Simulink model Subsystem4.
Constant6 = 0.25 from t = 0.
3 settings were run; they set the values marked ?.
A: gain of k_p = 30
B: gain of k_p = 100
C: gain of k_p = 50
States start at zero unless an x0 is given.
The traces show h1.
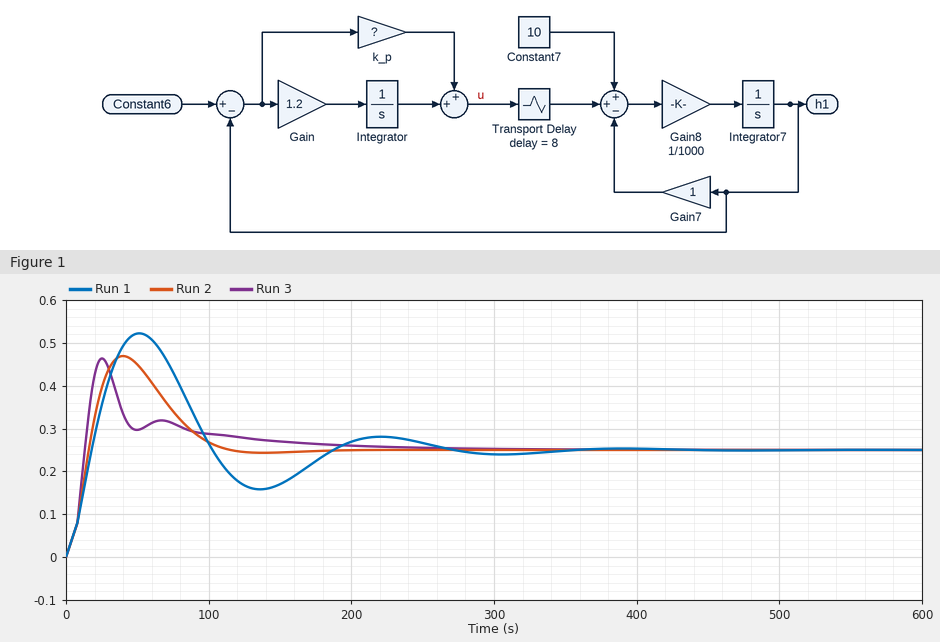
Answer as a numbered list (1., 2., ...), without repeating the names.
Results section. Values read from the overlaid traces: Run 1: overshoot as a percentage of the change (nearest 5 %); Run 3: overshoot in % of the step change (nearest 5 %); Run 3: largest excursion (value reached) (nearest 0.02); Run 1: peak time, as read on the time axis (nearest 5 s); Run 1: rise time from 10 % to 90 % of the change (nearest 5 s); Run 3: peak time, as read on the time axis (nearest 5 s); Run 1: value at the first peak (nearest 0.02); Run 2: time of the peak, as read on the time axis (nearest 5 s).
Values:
1. 110 %
2. 85 %
3. 0.46
4. 50 s
5. 15 s
6. 25 s
7. 0.52
8. 40 s
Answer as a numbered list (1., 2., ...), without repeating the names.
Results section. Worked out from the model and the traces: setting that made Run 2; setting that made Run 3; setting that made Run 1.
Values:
1. C
2. B
3. A
